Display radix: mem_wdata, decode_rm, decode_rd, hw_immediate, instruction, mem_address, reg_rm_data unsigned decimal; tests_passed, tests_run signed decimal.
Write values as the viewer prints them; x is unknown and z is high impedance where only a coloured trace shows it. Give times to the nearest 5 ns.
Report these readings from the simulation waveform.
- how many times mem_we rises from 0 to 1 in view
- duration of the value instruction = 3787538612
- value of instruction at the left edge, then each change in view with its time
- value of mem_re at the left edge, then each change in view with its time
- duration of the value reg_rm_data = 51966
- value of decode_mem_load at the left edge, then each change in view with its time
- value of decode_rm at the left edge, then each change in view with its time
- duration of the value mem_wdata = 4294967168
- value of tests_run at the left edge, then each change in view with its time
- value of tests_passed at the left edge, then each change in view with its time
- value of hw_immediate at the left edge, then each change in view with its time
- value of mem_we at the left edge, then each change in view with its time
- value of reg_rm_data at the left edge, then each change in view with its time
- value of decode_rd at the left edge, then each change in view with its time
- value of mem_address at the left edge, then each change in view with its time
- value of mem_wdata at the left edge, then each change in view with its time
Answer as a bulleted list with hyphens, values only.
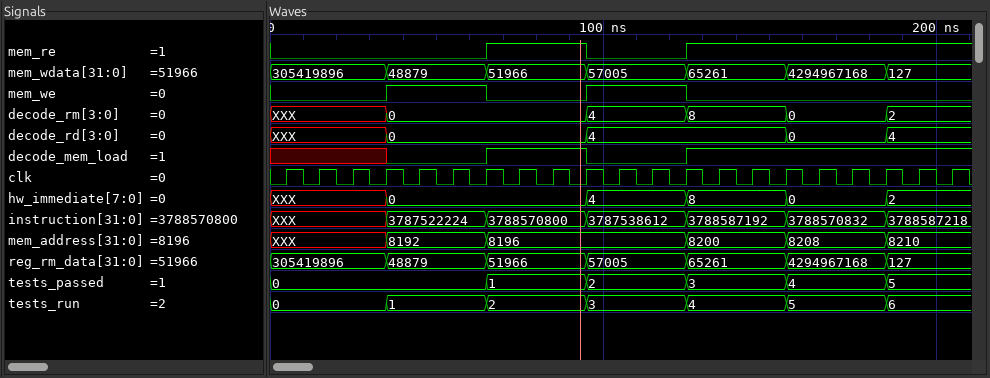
- 2
- 30 ns
- XXX, 3787522224 at 35 ns, 3788570800 at 65 ns, 3787538612 at 95 ns, 3788587192 at 125 ns, 3788570832 at 155 ns, 3788587218 at 185 ns
- 0, 1 at 65 ns, 0 at 95 ns, 1 at 125 ns
- 30 ns
- x, 0 at 35 ns, 1 at 65 ns, 0 at 95 ns, 1 at 125 ns
- XXX, 0 at 35 ns, 4 at 95 ns, 8 at 125 ns, 0 at 155 ns, 2 at 185 ns
- 30 ns
- 0, 1 at 35 ns, 2 at 65 ns, 3 at 95 ns, 4 at 125 ns, 5 at 155 ns, 6 at 185 ns
- 0, 1 at 65 ns, 2 at 95 ns, 3 at 125 ns, 4 at 155 ns, 5 at 185 ns
- XXX, 0 at 35 ns, 4 at 95 ns, 8 at 125 ns, 0 at 155 ns, 2 at 185 ns
- 0, 1 at 35 ns, 0 at 65 ns, 1 at 95 ns, 0 at 125 ns
- 305419896, 48879 at 35 ns, 51966 at 65 ns, 57005 at 95 ns, 65261 at 125 ns, 4294967168 at 155 ns, 127 at 185 ns
- XXX, 0 at 35 ns, 4 at 95 ns, 0 at 155 ns, 4 at 185 ns
- XXX, 8192 at 35 ns, 8196 at 65 ns, 8200 at 125 ns, 8208 at 155 ns, 8210 at 185 ns
- 305419896, 48879 at 35 ns, 51966 at 65 ns, 57005 at 95 ns, 65261 at 125 ns, 4294967168 at 155 ns, 127 at 185 ns
